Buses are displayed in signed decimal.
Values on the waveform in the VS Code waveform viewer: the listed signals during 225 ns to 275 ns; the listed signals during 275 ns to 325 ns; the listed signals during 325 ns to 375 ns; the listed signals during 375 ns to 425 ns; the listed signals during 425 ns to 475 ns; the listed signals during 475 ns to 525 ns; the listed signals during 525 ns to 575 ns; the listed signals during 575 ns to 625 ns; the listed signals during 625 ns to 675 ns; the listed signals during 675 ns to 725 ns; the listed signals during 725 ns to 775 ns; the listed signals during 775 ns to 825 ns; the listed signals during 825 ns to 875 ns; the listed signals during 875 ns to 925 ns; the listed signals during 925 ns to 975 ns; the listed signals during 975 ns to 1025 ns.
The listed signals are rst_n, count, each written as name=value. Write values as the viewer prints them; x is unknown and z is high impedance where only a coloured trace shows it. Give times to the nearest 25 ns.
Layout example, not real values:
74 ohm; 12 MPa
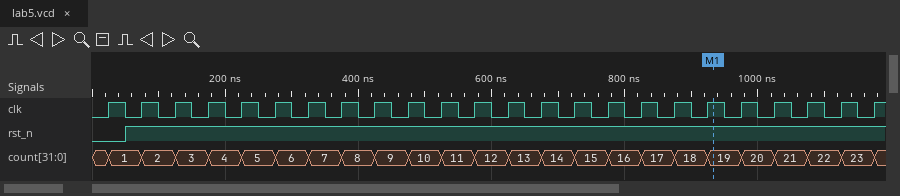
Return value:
rst_n=1, count=5; rst_n=1, count=6; rst_n=1, count=7; rst_n=1, count=8; rst_n=1, count=9; rst_n=1, count=10; rst_n=1, count=11; rst_n=1, count=12; rst_n=1, count=13; rst_n=1, count=14; rst_n=1, count=15; rst_n=1, count=16; rst_n=1, count=17; rst_n=1, count=18; rst_n=1, count=19; rst_n=1, count=20
